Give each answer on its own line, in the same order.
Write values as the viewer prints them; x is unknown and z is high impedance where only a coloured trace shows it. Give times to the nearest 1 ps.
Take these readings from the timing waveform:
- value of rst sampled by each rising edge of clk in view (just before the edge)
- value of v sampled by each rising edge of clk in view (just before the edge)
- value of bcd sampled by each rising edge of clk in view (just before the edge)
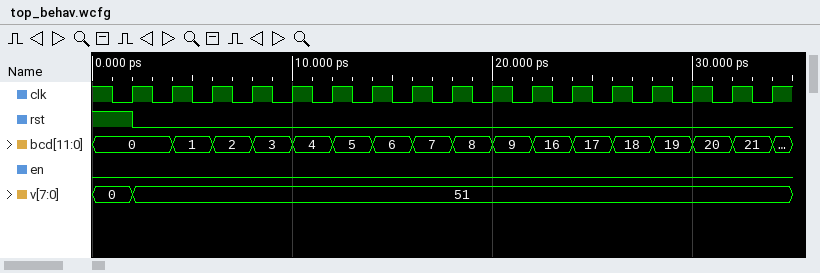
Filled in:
1 0 0 0 0 0 0 0 0 0 0 0 0 0 0 0 0
0, 51, 51, 51, 51, 51, 51, 51, 51, 51, 51, 51, 51, 51, 51, 51, 51
0, 0, 1, 2, 3, 4, 5, 6, 7, 8, 9, 16, 17, 18, 19, 20, 21
